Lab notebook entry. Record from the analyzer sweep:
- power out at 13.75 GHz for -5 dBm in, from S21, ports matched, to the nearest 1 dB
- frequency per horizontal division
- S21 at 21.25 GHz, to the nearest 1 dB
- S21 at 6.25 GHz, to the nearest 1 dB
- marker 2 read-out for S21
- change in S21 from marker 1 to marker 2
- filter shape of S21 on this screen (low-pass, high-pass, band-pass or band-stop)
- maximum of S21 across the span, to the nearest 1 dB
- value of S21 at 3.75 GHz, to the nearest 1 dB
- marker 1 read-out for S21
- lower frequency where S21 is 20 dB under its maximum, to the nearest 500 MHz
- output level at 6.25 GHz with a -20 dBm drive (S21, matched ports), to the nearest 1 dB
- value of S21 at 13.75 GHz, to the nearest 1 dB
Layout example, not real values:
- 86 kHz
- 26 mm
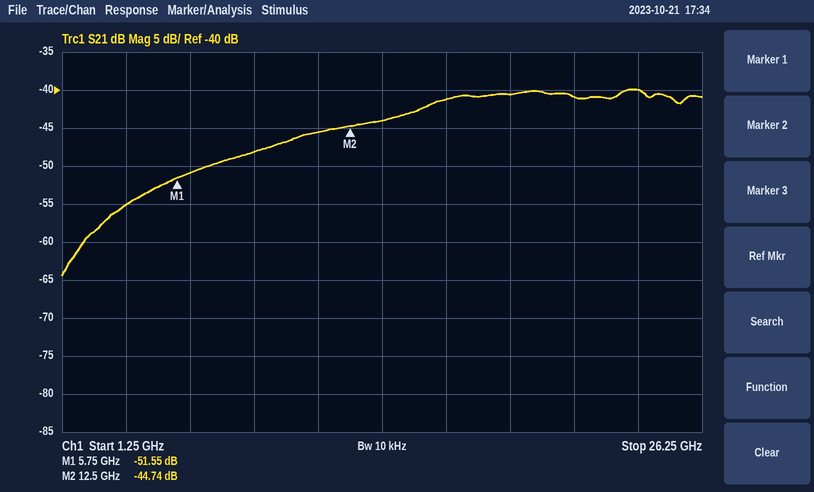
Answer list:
- -49 dBm
- 2.5 GHz
- -41 dB
- -51 dB
- -44.74 dB
- 6.81 dB
- high-pass
- -40 dB
- -55 dB
- -51.55 dB
- 2.0 GHz
- -71 dBm
- -44 dB
